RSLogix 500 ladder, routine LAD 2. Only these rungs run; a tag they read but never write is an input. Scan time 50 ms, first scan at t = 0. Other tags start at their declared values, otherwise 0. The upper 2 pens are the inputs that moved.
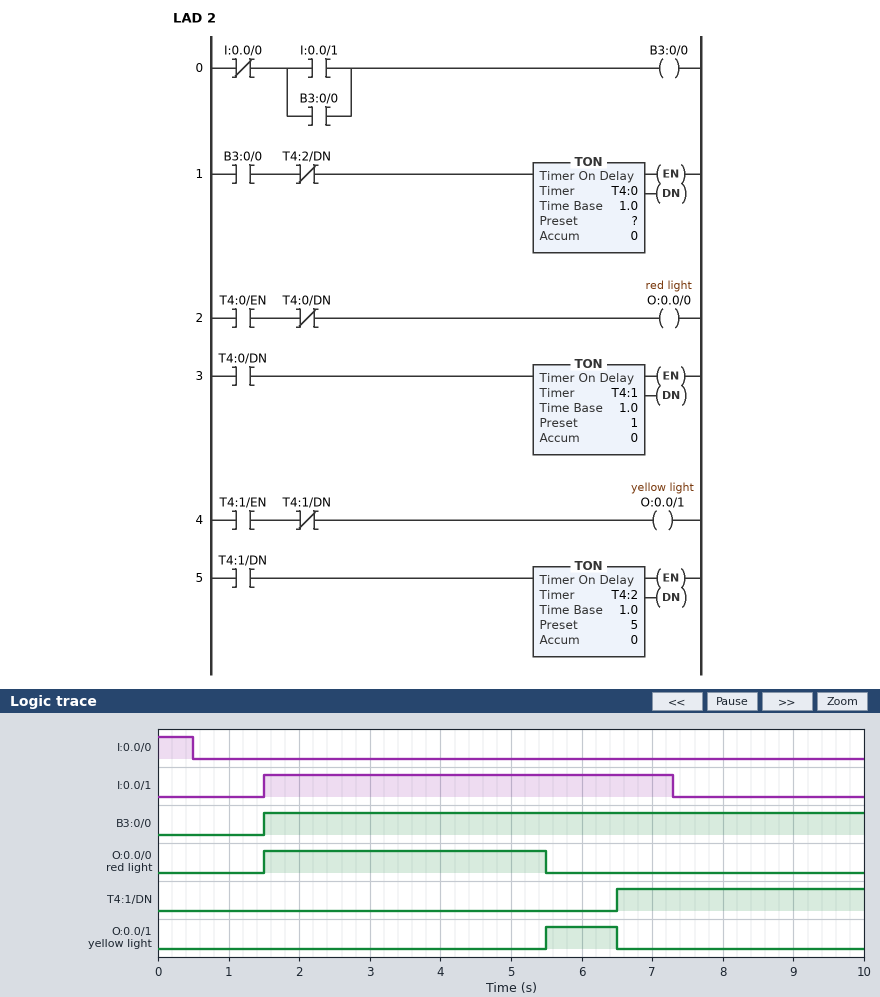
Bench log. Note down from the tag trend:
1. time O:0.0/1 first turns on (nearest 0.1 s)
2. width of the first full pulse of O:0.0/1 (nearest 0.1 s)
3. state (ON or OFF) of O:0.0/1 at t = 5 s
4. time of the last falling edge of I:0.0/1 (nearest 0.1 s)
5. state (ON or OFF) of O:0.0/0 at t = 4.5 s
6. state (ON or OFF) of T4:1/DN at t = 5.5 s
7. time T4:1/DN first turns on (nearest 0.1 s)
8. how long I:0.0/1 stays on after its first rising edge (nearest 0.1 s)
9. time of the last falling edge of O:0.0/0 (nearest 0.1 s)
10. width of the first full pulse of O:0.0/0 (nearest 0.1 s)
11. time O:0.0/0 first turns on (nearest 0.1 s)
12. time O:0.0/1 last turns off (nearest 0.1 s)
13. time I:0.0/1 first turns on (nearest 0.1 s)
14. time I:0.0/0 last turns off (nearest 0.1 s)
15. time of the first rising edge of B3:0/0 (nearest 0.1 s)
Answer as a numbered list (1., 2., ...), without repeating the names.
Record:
1. 5.5 s
2. 1.0 s
3. OFF
4. 7.3 s
5. ON
6. OFF
7. 6.5 s
8. 5.8 s
9. 5.5 s
10. 4.0 s
11. 1.5 s
12. 6.5 s
13. 1.5 s
14. 0.5 s
15. 1.5 s
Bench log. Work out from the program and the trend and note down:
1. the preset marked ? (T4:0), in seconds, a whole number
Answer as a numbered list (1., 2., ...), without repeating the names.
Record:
1. 4 s
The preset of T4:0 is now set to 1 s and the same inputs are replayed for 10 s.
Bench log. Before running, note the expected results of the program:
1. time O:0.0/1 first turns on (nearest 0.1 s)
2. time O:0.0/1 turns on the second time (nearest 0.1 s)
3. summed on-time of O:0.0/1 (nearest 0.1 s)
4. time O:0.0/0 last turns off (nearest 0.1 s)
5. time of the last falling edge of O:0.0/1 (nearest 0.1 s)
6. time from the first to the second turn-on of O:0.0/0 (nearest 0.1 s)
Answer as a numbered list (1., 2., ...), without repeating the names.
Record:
1. 2.5 s
2. 9.6 s
3. 1.4 s
4. 9.6 s
5. 3.5 s
6. 7.1 s
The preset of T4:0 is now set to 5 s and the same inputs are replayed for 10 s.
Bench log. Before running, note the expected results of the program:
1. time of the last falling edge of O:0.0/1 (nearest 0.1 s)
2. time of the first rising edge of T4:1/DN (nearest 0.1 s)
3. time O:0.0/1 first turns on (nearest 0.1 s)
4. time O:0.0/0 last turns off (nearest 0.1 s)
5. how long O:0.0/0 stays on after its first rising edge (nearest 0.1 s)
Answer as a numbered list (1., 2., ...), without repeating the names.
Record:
1. 7.5 s
2. 7.5 s
3. 6.5 s
4. 6.5 s
5. 5.0 s
